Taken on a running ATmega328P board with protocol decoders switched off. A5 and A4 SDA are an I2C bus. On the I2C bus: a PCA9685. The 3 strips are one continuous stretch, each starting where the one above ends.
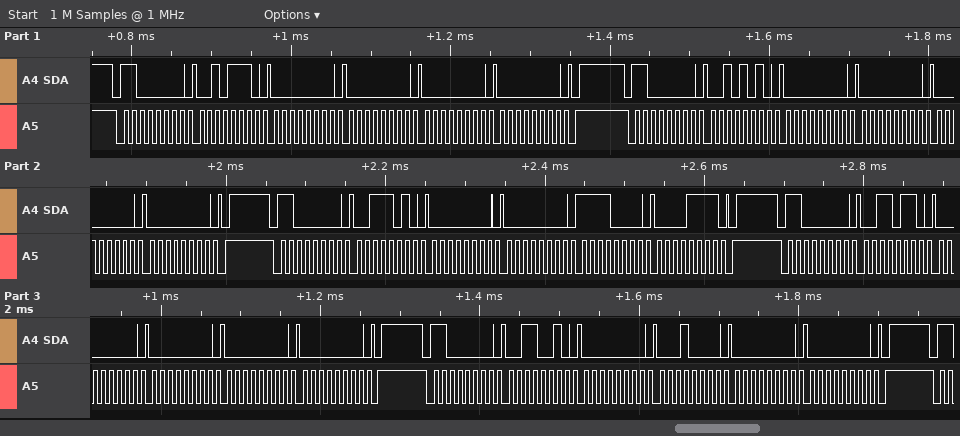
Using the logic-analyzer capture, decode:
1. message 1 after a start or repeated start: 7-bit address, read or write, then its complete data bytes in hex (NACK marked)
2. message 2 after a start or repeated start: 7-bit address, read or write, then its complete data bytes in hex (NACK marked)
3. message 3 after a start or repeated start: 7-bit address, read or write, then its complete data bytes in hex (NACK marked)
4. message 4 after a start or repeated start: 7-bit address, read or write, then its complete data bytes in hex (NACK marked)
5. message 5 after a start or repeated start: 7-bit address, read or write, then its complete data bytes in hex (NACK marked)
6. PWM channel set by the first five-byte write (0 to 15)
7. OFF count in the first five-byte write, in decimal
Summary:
0x60 write: 2E 00 00 00 00
0x60 write: 2A 00 00 00 00
0x60 write: 3A 00 00 F0 0F
0x60 write: 36 00 00 00 00
0x60 write: 32 00 10 00 00
10
0
